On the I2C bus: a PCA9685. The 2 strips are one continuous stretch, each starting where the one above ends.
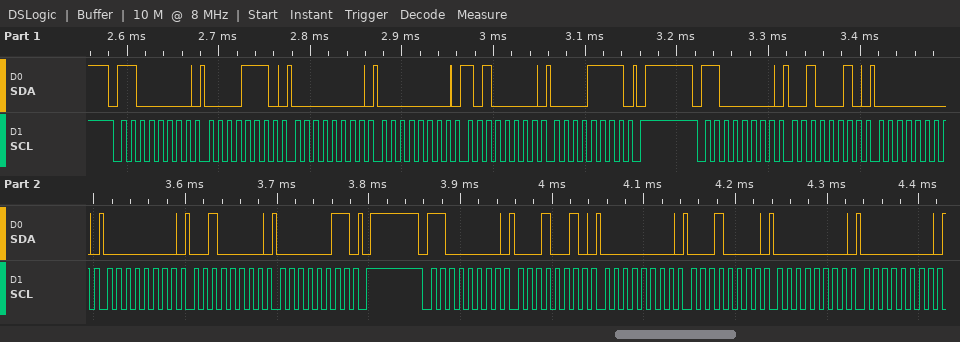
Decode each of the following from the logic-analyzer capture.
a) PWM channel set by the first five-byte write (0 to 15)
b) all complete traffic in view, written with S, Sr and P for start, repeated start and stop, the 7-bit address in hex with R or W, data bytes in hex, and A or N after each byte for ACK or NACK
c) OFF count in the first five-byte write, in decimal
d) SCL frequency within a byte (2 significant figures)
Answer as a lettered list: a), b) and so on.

a) 2
b) S 60W A 0E A 00 A 00 A A0 A 0F A P S 60W A 22 A 00 A 00 A 20 A 03 A P S 60W A 12 A 00 A 10 A 00 A 00 A
c) 4000
d) 100 kHz
